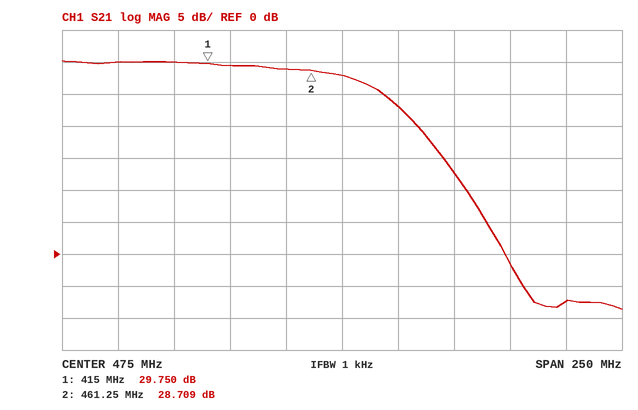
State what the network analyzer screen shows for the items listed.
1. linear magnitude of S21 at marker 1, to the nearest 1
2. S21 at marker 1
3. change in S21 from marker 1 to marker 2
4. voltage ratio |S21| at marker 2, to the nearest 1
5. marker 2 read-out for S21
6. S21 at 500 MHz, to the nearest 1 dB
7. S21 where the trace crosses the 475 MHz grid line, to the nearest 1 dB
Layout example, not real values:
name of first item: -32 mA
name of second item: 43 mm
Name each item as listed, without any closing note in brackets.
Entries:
linear magnitude of S21 at marker 1, to the nearest 1: 31
S21 at marker 1: 29.750 dB
change in S21 from marker 1 to marker 2: -1.041 dB
voltage ratio |S21| at marker 2, to the nearest 1: 27
marker 2 read-out for S21: 28.709 dB
S21 at 500 MHz, to the nearest 1 dB: 23 dB
S21 where the trace crosses the 475 MHz grid line, to the nearest 1 dB: 28 dB
